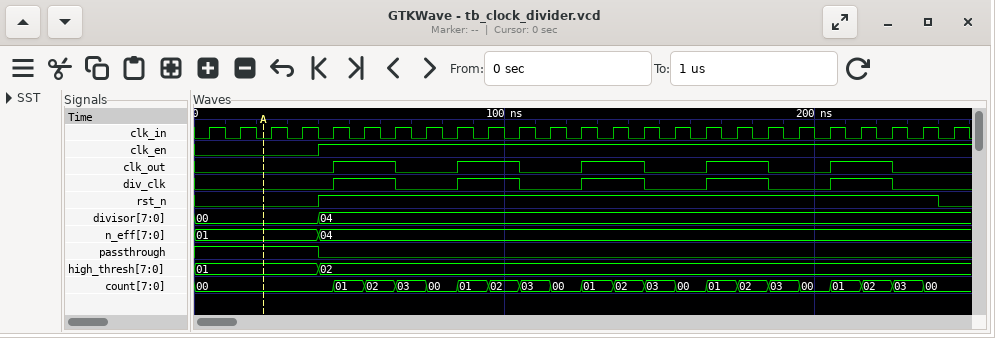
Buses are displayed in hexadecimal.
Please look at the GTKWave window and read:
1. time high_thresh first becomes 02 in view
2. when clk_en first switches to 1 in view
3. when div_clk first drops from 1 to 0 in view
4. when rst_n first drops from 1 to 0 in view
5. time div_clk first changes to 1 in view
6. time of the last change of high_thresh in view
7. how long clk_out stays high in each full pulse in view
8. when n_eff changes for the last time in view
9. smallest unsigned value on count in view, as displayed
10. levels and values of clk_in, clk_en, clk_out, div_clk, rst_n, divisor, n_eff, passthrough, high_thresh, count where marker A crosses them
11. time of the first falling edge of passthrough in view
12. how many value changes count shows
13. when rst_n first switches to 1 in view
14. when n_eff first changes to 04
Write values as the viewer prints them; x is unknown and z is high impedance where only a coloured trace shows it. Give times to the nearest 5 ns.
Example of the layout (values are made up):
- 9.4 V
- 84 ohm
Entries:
- 40 ns
- 40 ns
- 65 ns
- 240 ns
- 45 ns
- 40 ns
- 20 ns, 20 ns, 20 ns, 20 ns, 20 ns
- 40 ns
- 00
- clk_in=0, clk_en=0, clk_out=0, div_clk=0, rst_n=0, divisor=00, n_eff=01, passthrough=1, high_thresh=01, count=00
- 40 ns
- 20
- 40 ns
- 40 ns
